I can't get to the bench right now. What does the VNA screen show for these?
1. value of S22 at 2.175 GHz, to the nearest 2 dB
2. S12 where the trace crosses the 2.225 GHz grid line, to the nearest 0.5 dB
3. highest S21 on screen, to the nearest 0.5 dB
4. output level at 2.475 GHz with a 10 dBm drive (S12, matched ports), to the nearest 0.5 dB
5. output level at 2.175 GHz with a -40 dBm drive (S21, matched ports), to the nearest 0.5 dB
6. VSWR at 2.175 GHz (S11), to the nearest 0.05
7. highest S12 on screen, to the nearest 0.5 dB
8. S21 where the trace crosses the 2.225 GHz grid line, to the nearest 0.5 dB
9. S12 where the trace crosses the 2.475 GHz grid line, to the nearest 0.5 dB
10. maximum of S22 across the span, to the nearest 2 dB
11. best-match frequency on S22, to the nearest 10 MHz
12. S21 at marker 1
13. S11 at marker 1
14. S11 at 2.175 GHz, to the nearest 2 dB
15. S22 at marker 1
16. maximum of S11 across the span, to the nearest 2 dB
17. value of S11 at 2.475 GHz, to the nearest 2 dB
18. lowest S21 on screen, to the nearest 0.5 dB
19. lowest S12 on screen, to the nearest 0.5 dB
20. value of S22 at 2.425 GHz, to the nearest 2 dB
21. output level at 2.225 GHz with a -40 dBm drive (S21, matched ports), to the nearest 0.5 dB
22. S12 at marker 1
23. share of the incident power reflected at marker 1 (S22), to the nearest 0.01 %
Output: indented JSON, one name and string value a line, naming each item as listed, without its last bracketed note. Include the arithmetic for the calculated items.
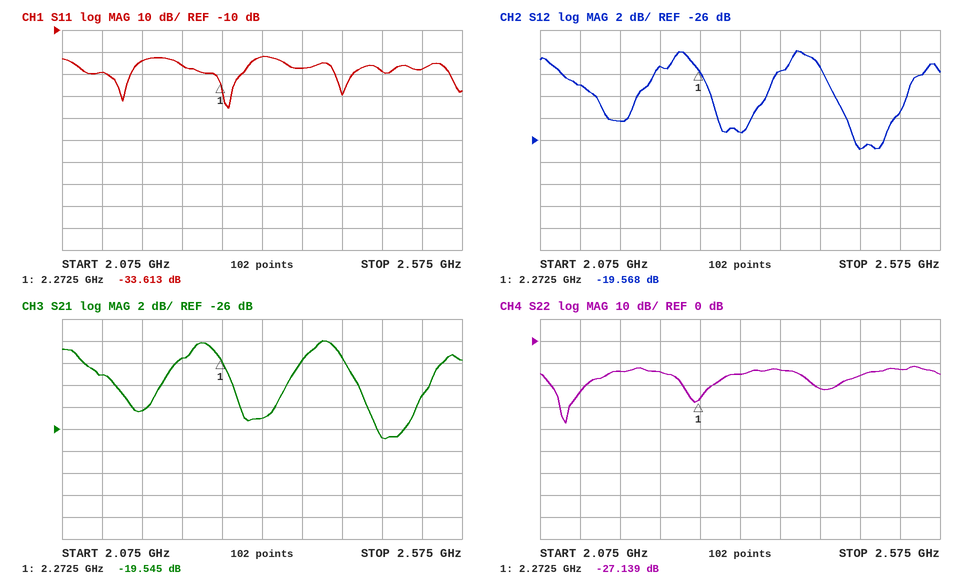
{
  "value of S22 at 2.175 GHz, to the nearest 2 dB": "-14 dB",
  "S12 where the trace crosses the 2.225 GHz grid line, to the nearest 0.5 dB": "-19.5 dB",
  "highest S21 on screen, to the nearest 0.5 dB": "-18.0 dB",
  "output level at 2.475 GHz with a 10 dBm drive (S12, matched ports), to the nearest 0.5 dB": "10 dBm + (-27.0 dB) = -17.0 dBm",
  "output level at 2.175 GHz with a -40 dBm drive (S21, matched ports), to the nearest 0.5 dB": "-40 dBm + (-24.5 dB) = -64.5 dBm",
  "VSWR at 2.175 GHz (S11), to the nearest 0.05": "|Γ| = 10^(-24/20) = 0.0631; VSWR = (1 + 0.0631)/(1 − 0.0631) ≈ 1.13, so 1.15 to the nearest 0.05",
  "highest S12 on screen, to the nearest 0.5 dB": "-18.0 dB",
  "S21 where the trace crosses the 2.225 GHz grid line, to the nearest 0.5 dB": "-19.5 dB",
  "S12 where the trace crosses the 2.475 GHz grid line, to the nearest 0.5 dB": "-27.0 dB",
  "maximum of S22 across the span, to the nearest 2 dB": "-12 dB",
  "best-match frequency on S22, to the nearest 10 MHz": "2.11 GHz",
  "S21 at marker 1": "-19.545 dB",
  "S11 at marker 1": "-33.613 dB",
  "S11 at 2.175 GHz, to the nearest 2 dB": "-24 dB",
  "S22 at marker 1": "-27.139 dB",
  "maximum of S11 across the span, to the nearest 2 dB": "-22 dB",
  "value of S11 at 2.475 GHz, to the nearest 2 dB": "-28 dB",
  "lowest S21 on screen, to the nearest 0.5 dB": "-27.0 dB",
  "lowest S12 on screen, to the nearest 0.5 dB": "-27.0 dB",
  "value of S22 at 2.425 GHz, to the nearest 2 dB": "-22 dB",
  "output level at 2.225 GHz with a -40 dBm drive (S21, matched ports), to the nearest 0.5 dB": "-40 dBm + (-19.5 dB) = -59.5 dBm",
  "S12 at marker 1": "-19.568 dB",
  "share of the incident power reflected at marker 1 (S22), to the nearest 0.01 %": "10^(-27.139/10) ≈ 0.19 %"
}
